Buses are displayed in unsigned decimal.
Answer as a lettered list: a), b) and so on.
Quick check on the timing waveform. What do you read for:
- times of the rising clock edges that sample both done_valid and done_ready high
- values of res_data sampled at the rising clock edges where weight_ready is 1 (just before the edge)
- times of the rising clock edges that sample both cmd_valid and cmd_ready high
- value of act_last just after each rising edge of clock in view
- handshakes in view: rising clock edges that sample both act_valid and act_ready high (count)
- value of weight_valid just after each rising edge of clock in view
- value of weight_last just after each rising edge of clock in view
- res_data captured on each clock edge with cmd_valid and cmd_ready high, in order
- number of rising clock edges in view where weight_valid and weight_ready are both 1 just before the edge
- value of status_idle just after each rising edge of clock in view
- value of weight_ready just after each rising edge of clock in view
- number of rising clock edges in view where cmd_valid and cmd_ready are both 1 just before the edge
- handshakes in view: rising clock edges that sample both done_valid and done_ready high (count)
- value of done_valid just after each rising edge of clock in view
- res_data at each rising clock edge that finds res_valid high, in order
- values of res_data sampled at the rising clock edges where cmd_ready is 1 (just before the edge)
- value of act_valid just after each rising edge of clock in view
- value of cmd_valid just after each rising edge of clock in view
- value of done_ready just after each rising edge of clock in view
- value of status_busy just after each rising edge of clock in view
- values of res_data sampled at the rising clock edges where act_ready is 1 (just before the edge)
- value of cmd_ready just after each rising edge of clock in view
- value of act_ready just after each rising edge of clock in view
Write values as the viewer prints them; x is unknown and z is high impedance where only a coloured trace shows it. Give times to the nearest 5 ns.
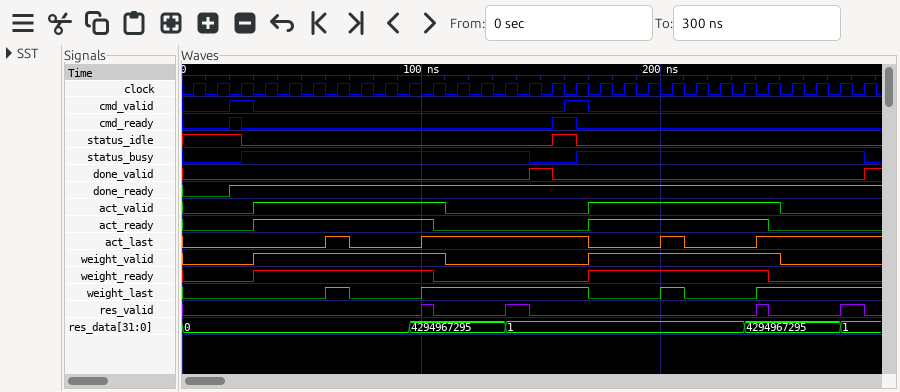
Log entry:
a) 155 ns
b) 0, 0, 0, 0, 0, 0, 0, 4294967295, 1, 1, 1, 1, 1, 1, 1, 4294967295
c) 25 ns, 165 ns
d) 0 0 0 0 0 0 1 0 0 0 1 1 1 1 1 1 1 0 0 0 1 0 0 0 1 1 1 1 1
e) 16
f) 0 0 0 1 1 1 1 1 1 1 1 0 0 0 0 0 0 1 1 1 1 1 1 1 1 0 0 0 0
g) 0 0 0 0 0 0 1 0 0 0 1 1 1 1 1 1 1 0 0 0 1 0 0 0 1 1 1 1 1
h) 0, 1
i) 16
j) 1 1 0 0 0 0 0 0 0 0 0 0 0 0 0 1 0 0 0 0 0 0 0 0 0 0 0 0 0
k) 0 0 0 1 1 1 1 1 1 1 0 0 0 0 0 0 0 1 1 1 1 1 1 1 0 0 0 0 0
l) 2
m) 1
n) 0 0 0 0 0 0 0 0 0 0 0 0 0 0 1 0 0 0 0 0 0 0 0 0 0 0 0 0 1
o) 4294967295, 1, 4294967295, 1
p) 0, 1
q) 0 0 0 1 1 1 1 1 1 1 1 0 0 0 0 0 0 1 1 1 1 1 1 1 1 0 0 0 0
r) 0 0 1 0 0 0 0 0 0 0 0 0 0 0 0 0 1 0 0 0 0 0 0 0 0 0 0 0 0
s) 0 0 1 1 1 1 1 1 1 1 1 1 1 1 1 1 1 1 1 1 1 1 1 1 1 1 1 1 1
t) 0 0 1 1 1 1 1 1 1 1 1 1 1 1 0 0 1 1 1 1 1 1 1 1 1 1 1 1 0
u) 0, 0, 0, 0, 0, 0, 0, 4294967295, 1, 1, 1, 1, 1, 1, 1, 4294967295
v) 0 0 0 0 0 0 0 0 0 0 0 0 0 0 0 1 0 0 0 0 0 0 0 0 0 0 0 0 0
w) 0 0 0 1 1 1 1 1 1 1 0 0 0 0 0 0 0 1 1 1 1 1 1 1 0 0 0 0 0
